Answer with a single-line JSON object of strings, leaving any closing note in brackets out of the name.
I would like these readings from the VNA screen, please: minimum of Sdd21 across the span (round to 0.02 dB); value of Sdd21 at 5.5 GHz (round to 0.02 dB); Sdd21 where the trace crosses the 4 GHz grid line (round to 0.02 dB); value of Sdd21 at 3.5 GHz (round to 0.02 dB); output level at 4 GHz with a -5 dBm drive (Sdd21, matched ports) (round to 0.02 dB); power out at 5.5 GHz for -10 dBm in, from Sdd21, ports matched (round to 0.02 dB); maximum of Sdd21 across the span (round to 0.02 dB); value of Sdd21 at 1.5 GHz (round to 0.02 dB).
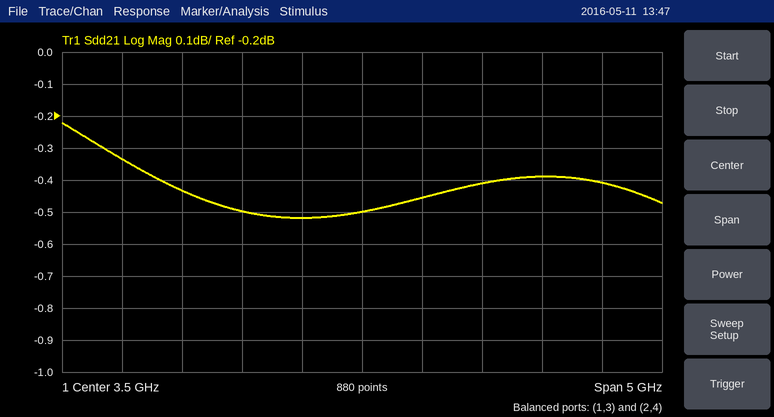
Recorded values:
{"minimum of Sdd21 across the span": "-0.52 dB", "value of Sdd21 at 5.5 GHz": "-0.40 dB", "Sdd21 where the trace crosses the 4 GHz grid line": "-0.46 dB", "value of Sdd21 at 3.5 GHz": "-0.50 dB", "output level at 4 GHz with a -5 dBm drive (Sdd21, matched ports)": "-5.46 dBm", "power out at 5.5 GHz for -10 dBm in, from Sdd21, ports matched": "-10.40 dBm", "maximum of Sdd21 across the span": "-0.22 dB", "value of Sdd21 at 1.5 GHz": "-0.34 dB"}
